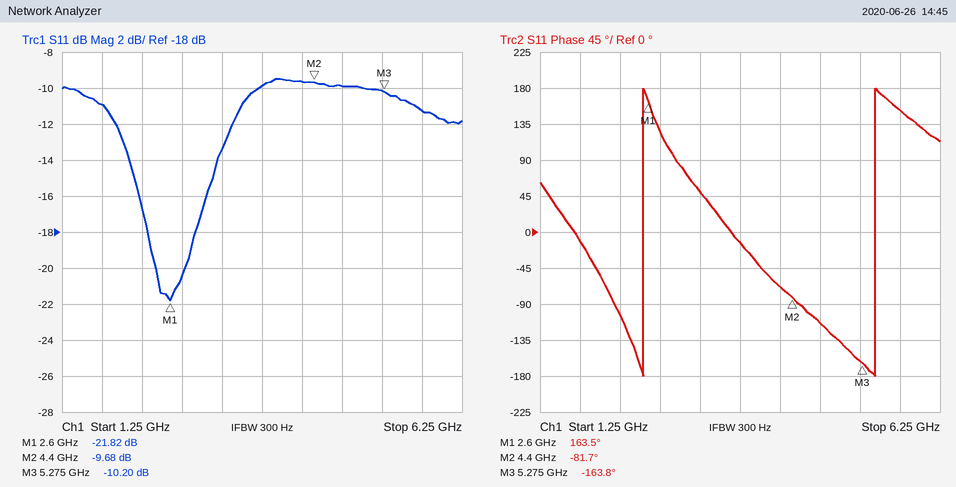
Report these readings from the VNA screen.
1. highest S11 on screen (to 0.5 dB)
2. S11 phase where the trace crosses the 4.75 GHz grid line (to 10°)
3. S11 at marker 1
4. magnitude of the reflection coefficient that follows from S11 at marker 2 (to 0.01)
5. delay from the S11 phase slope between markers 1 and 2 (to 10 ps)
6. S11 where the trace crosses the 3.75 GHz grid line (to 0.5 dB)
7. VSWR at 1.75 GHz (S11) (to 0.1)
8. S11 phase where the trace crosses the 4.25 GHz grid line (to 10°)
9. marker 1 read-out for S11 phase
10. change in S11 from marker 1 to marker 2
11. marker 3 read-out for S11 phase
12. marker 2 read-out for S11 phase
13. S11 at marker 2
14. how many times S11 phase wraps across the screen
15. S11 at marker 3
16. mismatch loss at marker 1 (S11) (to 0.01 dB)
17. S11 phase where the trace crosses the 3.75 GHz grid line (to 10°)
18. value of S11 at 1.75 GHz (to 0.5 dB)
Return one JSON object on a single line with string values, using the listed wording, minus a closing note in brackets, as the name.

{"highest S11 on screen": "-9.5 dB", "S11 phase where the trace crosses the 4.75 GHz grid line": "-110°", "S11 at marker 1": "-21.82 dB", "magnitude of the reflection coefficient that follows from S11 at marker 2": "0.33", "delay from the S11 phase slope between markers 1 and 2": "380 ps", "S11 where the trace crosses the 3.75 GHz grid line": "-10.0 dB", "VSWR at 1.75 GHz (S11)": "1.8", "S11 phase where the trace crosses the 4.25 GHz grid line": "-70°", "marker 1 read-out for S11 phase": "163.5°", "change in S11 from marker 1 to marker 2": "12.14 dB", "marker 3 read-out for S11 phase": "-163.8°", "marker 2 read-out for S11 phase": "-81.7°", "S11 at marker 2": "-9.68 dB", "how many times S11 phase wraps across the screen": "2", "S11 at marker 3": "-10.20 dB", "mismatch loss at marker 1 (S11)": "0.03 dB", "S11 phase where the trace crosses the 3.75 GHz grid line": "-10°", "value of S11 at 1.75 GHz": "-11.0 dB"}
